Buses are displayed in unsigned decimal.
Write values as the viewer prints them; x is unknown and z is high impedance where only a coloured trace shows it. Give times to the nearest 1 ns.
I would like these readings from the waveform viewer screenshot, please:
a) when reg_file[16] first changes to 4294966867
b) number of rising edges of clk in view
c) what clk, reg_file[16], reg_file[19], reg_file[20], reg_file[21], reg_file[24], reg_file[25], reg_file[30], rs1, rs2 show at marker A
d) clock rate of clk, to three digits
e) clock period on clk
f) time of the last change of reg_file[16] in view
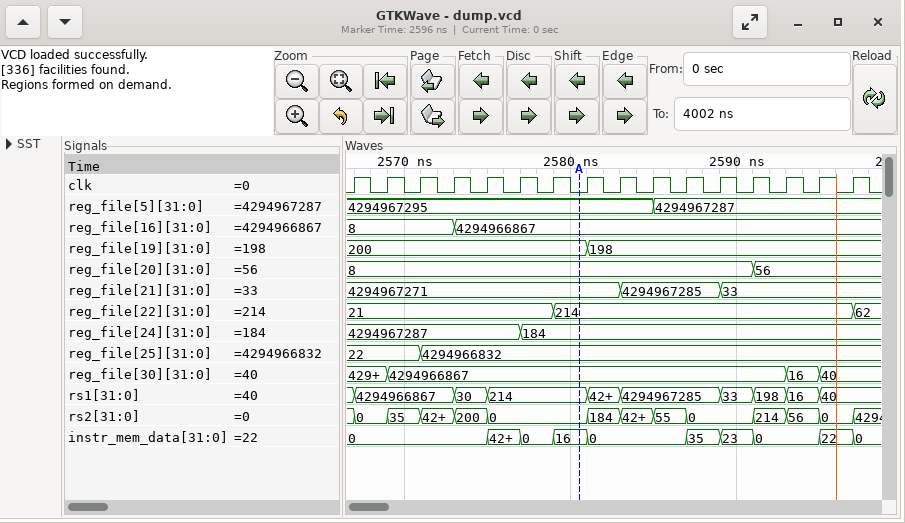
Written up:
2573 ns
16
clk=0, reg_file[16]=4294966867, reg_file[19]=200, reg_file[20]=8, reg_file[21]=4294967271, reg_file[24]=184, reg_file[25]=4294966832, reg_file[30]=4294966867, rs1=214, rs2=0
500 MHz
2 ns
2573 ns
